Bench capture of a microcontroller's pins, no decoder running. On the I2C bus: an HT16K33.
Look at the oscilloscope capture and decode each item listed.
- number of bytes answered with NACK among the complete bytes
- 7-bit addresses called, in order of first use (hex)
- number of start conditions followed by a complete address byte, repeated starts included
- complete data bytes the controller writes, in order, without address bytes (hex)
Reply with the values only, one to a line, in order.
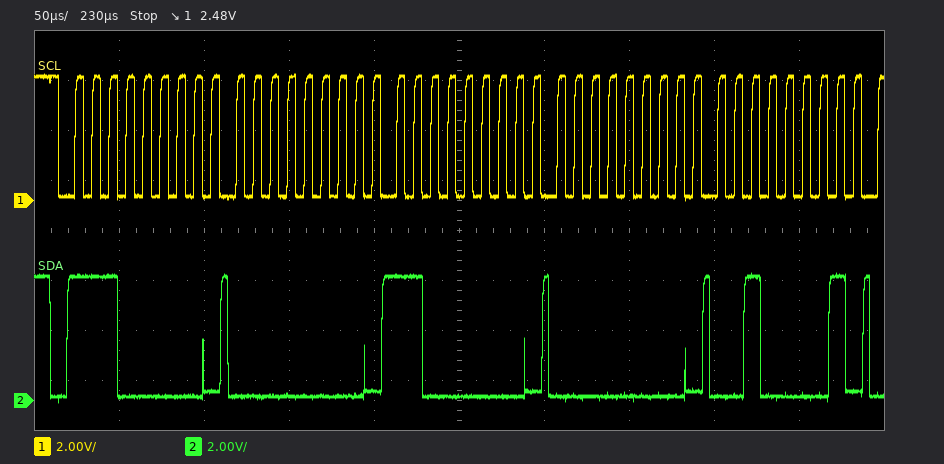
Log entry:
0
0x70
1
00 C0 00 21
